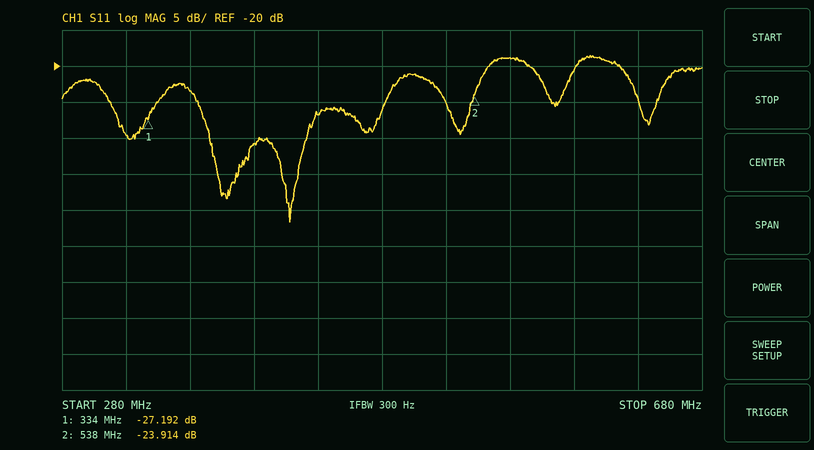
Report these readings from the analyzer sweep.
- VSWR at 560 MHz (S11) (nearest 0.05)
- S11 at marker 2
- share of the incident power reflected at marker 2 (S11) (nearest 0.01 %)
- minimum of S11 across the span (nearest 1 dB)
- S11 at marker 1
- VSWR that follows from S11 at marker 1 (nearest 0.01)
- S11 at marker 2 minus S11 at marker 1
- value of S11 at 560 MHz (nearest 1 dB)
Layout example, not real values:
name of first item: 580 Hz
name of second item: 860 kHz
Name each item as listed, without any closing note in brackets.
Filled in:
VSWR at 560 MHz (S11): 1.25
S11 at marker 2: -23.914 dB
share of the incident power reflected at marker 2 (S11): 0.41 %
minimum of S11 across the span: -42 dB
S11 at marker 1: -27.192 dB
VSWR that follows from S11 at marker 1: 1.09
S11 at marker 2 minus S11 at marker 1: 3.278 dB
value of S11 at 560 MHz: -19 dB
